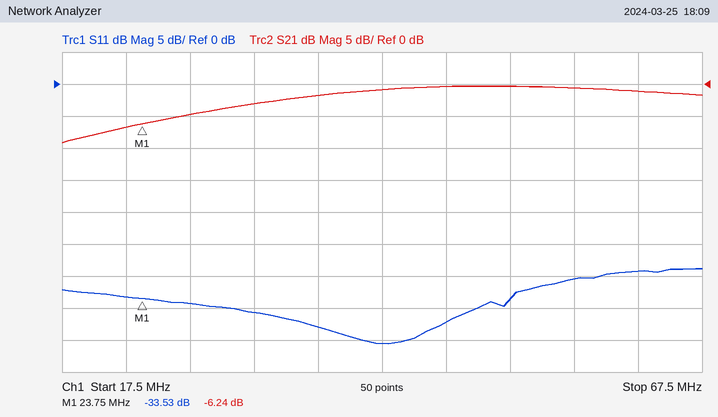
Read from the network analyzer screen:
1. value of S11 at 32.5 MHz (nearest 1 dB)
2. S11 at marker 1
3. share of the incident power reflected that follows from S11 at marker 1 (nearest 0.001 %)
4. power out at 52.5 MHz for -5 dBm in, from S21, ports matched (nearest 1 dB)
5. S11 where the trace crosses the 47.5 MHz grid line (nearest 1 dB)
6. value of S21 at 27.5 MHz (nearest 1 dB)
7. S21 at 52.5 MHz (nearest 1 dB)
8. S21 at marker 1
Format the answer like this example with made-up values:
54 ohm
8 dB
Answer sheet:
-36 dB
-33.53 dB
0.044 %
-5 dBm
-37 dB
-5 dB
0 dB
-6.24 dB
